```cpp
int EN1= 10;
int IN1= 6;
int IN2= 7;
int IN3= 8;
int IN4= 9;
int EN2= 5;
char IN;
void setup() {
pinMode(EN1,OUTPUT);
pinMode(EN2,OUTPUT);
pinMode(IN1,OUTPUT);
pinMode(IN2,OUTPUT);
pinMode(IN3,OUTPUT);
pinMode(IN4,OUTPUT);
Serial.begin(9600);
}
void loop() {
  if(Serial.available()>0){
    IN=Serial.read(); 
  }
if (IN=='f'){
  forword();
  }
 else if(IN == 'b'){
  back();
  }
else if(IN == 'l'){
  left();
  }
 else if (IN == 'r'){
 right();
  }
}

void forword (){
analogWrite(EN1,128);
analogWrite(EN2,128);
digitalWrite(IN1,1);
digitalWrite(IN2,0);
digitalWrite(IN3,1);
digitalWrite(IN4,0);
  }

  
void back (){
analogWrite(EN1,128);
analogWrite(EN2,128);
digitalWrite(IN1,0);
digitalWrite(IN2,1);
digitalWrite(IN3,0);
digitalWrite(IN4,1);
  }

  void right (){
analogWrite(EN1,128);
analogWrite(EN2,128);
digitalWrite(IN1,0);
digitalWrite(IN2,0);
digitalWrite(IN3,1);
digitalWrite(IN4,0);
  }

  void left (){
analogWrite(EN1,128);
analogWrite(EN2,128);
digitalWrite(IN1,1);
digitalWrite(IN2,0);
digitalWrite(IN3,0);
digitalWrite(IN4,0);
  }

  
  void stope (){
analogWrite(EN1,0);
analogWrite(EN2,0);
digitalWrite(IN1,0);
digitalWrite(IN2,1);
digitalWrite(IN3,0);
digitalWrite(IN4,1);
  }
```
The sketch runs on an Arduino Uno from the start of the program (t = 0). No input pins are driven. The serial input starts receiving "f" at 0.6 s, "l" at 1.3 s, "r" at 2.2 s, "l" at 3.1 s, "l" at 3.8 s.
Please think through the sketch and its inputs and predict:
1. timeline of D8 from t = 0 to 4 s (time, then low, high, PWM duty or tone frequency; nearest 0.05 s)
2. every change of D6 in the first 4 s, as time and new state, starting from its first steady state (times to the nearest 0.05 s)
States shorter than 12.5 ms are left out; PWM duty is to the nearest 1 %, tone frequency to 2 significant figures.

0 s low; 0.6 s high; 1.3 s low; 2.2 s high; 3.1 s low
0 s low; 0.6 s high; 2.2 s low; 3.1 s high
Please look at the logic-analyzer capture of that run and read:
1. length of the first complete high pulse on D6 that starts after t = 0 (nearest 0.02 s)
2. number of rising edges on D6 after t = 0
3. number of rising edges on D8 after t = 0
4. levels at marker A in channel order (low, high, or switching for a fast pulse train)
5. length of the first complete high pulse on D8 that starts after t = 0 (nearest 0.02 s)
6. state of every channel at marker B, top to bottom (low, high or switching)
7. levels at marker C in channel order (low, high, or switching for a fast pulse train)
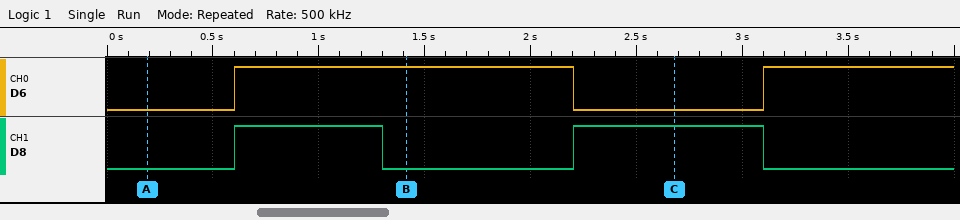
1.60 s
2
2
D6 low, D8 low
0.70 s
D6 high, D8 low
D6 low, D8 high
